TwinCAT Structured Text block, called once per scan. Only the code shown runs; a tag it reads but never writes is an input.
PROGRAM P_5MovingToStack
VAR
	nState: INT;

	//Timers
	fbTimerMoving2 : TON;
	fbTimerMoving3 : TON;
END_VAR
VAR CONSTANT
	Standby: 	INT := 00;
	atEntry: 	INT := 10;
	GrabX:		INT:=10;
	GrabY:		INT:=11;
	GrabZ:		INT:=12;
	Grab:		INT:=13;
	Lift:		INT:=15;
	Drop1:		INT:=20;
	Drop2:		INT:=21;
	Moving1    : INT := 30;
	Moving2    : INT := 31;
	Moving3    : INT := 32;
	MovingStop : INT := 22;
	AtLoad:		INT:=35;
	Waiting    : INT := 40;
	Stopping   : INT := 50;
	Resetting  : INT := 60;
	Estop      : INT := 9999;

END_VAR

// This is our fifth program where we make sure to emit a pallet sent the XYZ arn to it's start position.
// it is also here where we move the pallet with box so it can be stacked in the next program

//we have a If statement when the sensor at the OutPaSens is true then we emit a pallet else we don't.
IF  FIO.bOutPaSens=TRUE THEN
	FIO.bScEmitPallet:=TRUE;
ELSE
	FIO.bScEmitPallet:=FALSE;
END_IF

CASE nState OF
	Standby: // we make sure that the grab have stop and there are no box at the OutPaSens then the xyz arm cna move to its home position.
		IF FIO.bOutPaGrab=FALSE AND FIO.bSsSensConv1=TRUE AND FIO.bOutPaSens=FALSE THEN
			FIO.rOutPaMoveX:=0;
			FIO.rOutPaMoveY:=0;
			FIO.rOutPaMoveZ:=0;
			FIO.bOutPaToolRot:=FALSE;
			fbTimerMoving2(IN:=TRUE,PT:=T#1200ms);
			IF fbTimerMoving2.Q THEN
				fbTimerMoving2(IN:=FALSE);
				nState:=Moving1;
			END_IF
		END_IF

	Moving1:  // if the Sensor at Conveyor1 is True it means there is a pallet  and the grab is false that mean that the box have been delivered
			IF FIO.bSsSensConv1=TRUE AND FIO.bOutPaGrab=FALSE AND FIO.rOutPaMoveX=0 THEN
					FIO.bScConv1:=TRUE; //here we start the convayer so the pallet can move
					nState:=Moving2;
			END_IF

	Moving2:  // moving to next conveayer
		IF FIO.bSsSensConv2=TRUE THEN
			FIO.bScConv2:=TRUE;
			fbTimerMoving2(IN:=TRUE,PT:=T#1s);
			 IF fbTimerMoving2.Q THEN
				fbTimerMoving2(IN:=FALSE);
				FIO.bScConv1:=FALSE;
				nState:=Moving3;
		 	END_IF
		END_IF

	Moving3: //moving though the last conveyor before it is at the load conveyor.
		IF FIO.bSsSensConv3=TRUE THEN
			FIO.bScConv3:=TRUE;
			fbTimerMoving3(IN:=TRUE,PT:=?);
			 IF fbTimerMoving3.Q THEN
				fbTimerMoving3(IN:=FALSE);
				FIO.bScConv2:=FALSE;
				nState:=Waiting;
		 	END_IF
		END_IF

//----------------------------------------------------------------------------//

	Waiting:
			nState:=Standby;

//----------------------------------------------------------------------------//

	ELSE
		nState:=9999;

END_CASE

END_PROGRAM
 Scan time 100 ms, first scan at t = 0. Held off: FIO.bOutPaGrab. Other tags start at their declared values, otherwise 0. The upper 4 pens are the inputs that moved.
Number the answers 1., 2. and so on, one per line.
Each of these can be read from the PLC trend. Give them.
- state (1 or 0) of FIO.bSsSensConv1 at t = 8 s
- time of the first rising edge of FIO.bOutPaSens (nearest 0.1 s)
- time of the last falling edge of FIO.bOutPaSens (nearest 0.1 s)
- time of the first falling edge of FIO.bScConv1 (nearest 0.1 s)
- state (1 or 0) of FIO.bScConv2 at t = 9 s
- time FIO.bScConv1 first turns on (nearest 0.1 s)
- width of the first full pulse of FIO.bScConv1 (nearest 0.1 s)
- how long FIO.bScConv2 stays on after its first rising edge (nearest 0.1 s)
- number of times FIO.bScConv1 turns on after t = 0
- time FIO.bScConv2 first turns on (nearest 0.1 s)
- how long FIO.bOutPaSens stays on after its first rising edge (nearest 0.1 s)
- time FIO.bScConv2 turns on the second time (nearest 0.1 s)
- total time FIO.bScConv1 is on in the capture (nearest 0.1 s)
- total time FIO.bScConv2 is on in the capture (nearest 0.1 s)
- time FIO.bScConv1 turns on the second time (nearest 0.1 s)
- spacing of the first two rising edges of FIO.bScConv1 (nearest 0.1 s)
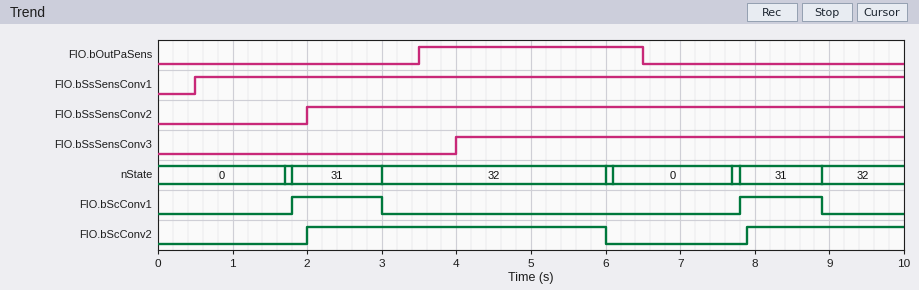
1. 1
2. 3.5 s
3. 6.5 s
4. 3.0 s
5. 1
6. 1.8 s
7. 1.2 s
8. 4.0 s
9. 2
10. 2.0 s
11. 3.0 s
12. 7.9 s
13. 2.3 s
14. 6.1 s
15. 7.8 s
16. 6.0 s
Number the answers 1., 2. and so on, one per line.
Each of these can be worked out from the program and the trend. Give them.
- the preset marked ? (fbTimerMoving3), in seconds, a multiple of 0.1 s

1. 2.0 s
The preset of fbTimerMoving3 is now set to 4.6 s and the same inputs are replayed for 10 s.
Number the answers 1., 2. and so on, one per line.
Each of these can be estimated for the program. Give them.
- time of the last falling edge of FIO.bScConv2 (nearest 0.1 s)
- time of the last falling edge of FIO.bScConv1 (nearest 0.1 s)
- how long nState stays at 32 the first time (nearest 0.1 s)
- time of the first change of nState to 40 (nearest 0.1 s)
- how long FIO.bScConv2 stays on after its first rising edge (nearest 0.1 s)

1. 8.6 s
2. 3.0 s
3. 5.6 s
4. 8.6 s
5. 6.6 s
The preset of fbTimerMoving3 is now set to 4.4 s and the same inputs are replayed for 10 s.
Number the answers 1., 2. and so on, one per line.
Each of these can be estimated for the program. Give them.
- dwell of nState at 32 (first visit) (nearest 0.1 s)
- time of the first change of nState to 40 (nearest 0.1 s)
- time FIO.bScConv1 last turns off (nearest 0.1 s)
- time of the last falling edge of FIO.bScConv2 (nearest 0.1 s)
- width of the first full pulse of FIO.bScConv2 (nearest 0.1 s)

1. 5.4 s
2. 8.4 s
3. 3.0 s
4. 8.4 s
5. 6.4 s
